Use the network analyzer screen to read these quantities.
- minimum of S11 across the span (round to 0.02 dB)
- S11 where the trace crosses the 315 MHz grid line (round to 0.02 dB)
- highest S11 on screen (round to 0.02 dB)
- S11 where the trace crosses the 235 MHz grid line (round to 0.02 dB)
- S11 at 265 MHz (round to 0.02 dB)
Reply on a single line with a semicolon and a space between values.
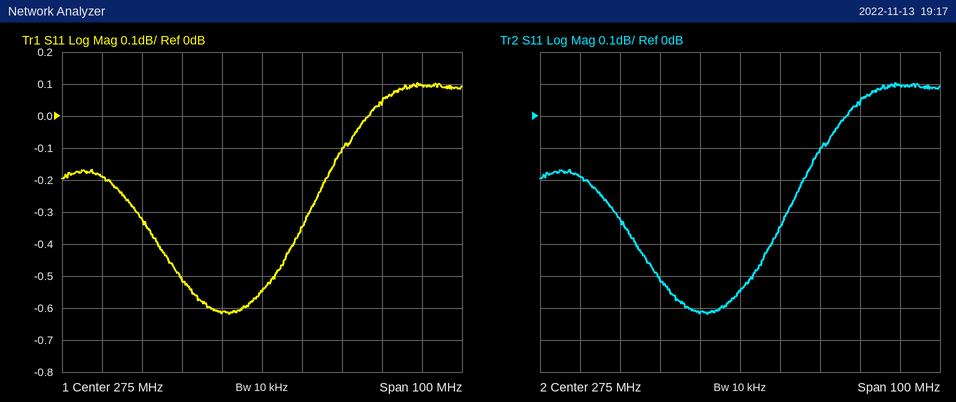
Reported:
-0.62 dB; 0.10 dB; 0.10 dB; -0.18 dB; -0.62 dB
